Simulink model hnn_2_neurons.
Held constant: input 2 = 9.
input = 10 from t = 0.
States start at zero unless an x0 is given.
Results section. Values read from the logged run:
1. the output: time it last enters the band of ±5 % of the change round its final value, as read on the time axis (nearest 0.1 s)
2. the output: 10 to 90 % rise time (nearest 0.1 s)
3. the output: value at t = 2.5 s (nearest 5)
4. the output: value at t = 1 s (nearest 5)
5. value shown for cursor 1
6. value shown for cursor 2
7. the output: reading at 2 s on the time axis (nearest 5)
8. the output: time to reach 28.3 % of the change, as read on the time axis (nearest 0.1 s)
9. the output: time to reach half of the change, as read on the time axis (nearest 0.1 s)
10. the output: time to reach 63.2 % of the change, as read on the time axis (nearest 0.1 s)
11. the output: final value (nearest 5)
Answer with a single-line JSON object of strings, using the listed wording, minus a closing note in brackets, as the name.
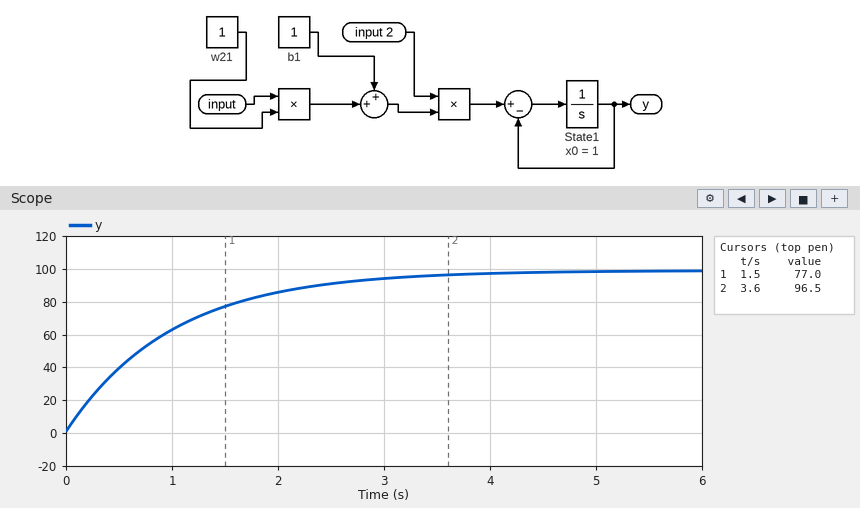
{"the output: time it last enters the band of ±5 % of the change round its final value, as read on the time axis": "3.0 s", "the output: 10 to 90 % rise time": "2.2 s", "the output: value at t = 2.5 s": "90", "the output: value at t = 1 s": "65", "value shown for cursor 1": "77.0", "value shown for cursor 2": "96.5", "the output: reading at 2 s on the time axis": "85", "the output: time to reach 28.3 % of the change, as read on the time axis": "0.3 s", "the output: time to reach half of the change, as read on the time axis": "0.7 s", "the output: time to reach 63.2 % of the change, as read on the time axis": "1.0 s", "the output: final value": "100"}
